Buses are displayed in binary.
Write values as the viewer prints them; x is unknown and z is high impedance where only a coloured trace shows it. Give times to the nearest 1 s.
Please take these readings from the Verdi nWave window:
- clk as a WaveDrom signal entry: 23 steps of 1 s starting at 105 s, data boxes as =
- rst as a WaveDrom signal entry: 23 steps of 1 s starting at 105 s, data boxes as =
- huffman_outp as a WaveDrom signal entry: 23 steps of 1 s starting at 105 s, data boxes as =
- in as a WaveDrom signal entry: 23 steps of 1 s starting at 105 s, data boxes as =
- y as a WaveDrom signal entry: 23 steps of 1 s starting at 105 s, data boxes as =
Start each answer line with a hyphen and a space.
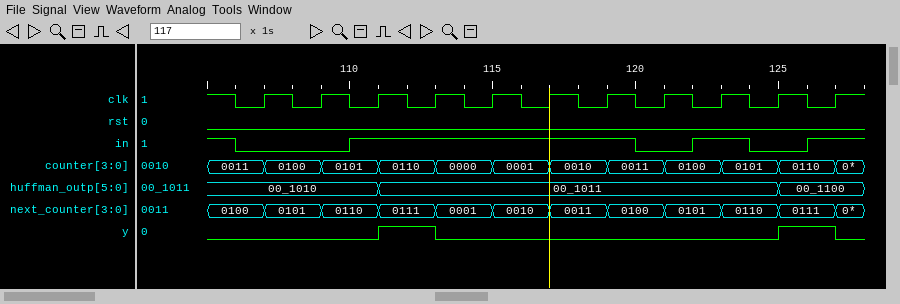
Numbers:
- {name: 'clk', wave: '10101010101010101010101'}
- {name: 'rst', wave: '0......................'}
- {name: 'huffman_outp', wave: '=.....=.............=..', data: '00_1010 00_1011 00_1100'}
- {name: 'in', wave: '10...1.........0.1.0.1.'}
- {name: 'y', wave: '0.....1.0...........1.0'}
